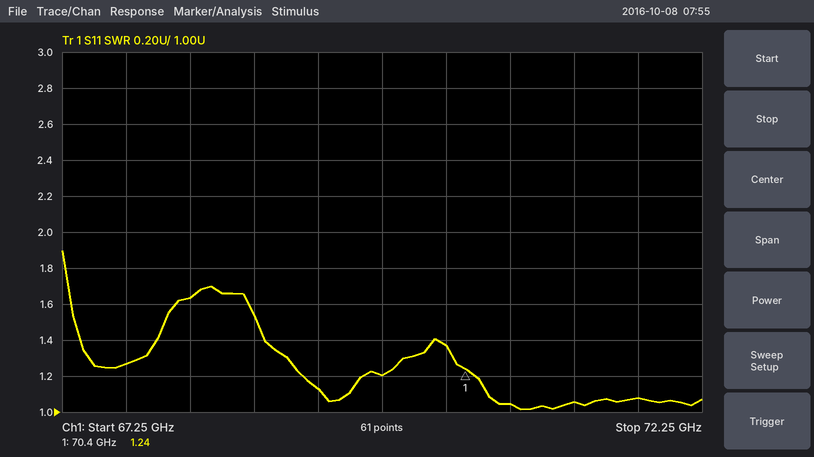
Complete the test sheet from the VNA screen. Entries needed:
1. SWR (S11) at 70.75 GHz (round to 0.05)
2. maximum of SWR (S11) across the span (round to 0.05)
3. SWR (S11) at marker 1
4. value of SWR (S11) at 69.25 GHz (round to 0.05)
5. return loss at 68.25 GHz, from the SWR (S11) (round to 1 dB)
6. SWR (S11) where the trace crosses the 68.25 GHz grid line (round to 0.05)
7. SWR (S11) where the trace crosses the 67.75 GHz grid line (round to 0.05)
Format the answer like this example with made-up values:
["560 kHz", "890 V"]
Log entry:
["1.05", "1.90", "1.24", "1.15", "12 dB", "1.65", "1.25"]
